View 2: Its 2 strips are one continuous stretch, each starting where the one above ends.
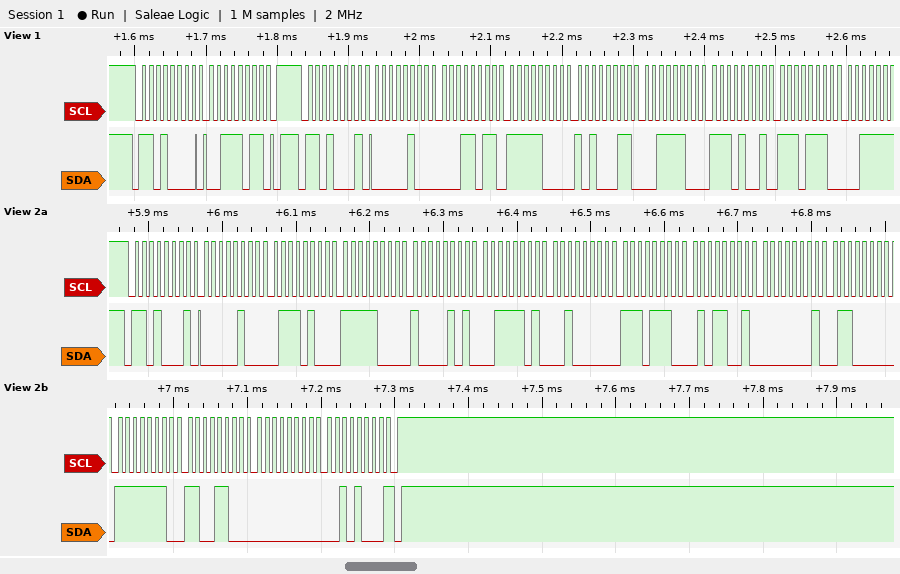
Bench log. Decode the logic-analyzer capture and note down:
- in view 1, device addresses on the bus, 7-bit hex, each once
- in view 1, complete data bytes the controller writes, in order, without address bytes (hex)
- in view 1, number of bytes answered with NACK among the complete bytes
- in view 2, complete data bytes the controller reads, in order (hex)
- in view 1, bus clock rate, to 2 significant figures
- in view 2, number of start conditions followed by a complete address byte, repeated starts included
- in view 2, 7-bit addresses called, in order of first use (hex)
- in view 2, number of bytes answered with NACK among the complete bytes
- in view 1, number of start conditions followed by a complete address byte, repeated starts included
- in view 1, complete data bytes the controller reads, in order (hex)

0x68
3B
0
04 74 F8 85 3D 20 EE 59 01 60 FE CC 00 28
100 kHz
1
0x68
1
2
04 1B F8 A3 3C E9 EE
